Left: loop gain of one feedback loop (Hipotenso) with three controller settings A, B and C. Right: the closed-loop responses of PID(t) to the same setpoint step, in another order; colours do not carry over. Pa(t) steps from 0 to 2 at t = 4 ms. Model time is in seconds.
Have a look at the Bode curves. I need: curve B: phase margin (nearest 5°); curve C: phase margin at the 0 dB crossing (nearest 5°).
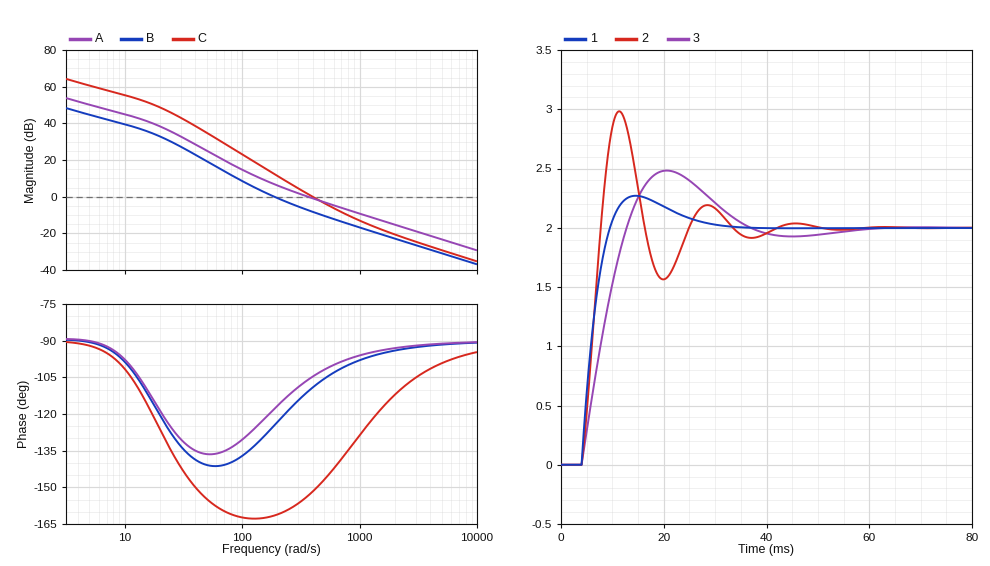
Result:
55°
30°
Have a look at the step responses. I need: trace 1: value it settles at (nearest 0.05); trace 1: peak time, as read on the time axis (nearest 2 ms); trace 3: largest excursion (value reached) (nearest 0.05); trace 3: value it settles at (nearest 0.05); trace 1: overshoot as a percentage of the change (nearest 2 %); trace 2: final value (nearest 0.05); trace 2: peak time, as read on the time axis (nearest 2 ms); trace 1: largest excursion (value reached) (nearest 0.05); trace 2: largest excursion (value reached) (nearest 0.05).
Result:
2.00
14 ms
2.50
2.00
14 %
2.00
12 ms
2.25
3.00
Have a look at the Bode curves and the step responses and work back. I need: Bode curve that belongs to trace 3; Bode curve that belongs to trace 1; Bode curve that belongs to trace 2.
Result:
B
A
C
